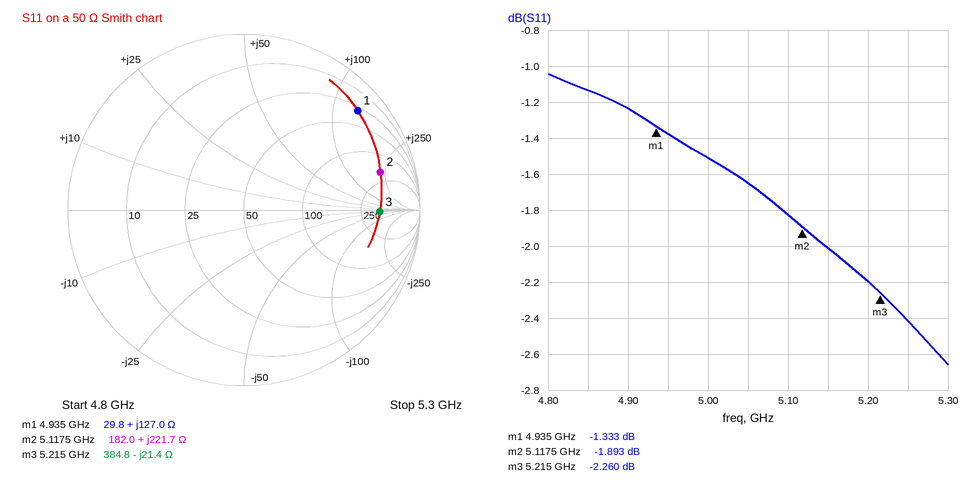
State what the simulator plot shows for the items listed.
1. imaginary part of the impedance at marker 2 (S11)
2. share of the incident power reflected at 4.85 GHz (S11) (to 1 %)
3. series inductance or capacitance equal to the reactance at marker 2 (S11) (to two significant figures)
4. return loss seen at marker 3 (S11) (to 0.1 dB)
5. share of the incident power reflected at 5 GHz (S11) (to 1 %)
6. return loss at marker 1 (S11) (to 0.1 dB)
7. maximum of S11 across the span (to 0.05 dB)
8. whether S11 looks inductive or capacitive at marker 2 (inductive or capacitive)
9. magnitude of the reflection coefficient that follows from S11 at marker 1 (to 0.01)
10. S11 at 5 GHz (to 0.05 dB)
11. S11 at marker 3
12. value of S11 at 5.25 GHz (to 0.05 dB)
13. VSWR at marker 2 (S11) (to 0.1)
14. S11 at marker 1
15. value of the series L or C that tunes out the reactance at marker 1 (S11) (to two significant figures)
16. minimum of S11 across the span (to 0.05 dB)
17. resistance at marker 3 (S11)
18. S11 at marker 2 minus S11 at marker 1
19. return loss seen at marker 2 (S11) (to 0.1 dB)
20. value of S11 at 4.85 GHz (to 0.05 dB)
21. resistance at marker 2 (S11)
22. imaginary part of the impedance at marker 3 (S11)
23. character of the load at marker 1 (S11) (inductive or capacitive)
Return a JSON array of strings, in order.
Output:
["+221.7 Ω", "77 %", "6.9 nH", "2.3 dB", "71 %", "1.3 dB", "-1.05 dB", "inductive", "0.86", "-1.50 dB", "-2.260 dB", "-2.40 dB", "9.2", "-1.333 dB", "250 fF", "-2.65 dB", "384.8 Ω", "-0.560 dB", "1.9 dB", "-1.15 dB", "182.0 Ω", "-21.4 Ω", "inductive"]
